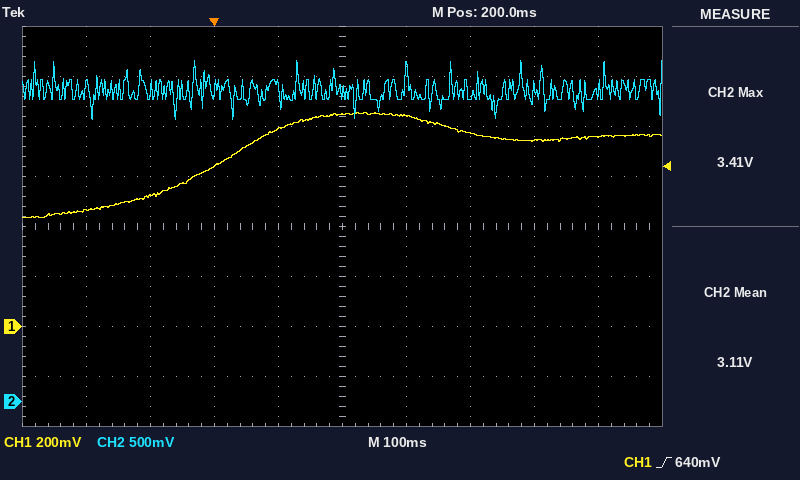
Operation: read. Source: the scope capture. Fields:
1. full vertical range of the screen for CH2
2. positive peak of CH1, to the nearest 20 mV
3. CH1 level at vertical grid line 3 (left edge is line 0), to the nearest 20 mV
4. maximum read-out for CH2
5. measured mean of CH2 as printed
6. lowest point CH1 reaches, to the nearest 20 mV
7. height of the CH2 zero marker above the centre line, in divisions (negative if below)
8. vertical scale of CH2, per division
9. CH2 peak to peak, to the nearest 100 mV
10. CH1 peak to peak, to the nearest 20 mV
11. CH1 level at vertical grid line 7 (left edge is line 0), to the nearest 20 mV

4 V
860 mV
640 mV
3.41 V
3.11 V
440 mV
-3.5 div
500 mV
600 mV
420 mV
780 mV
